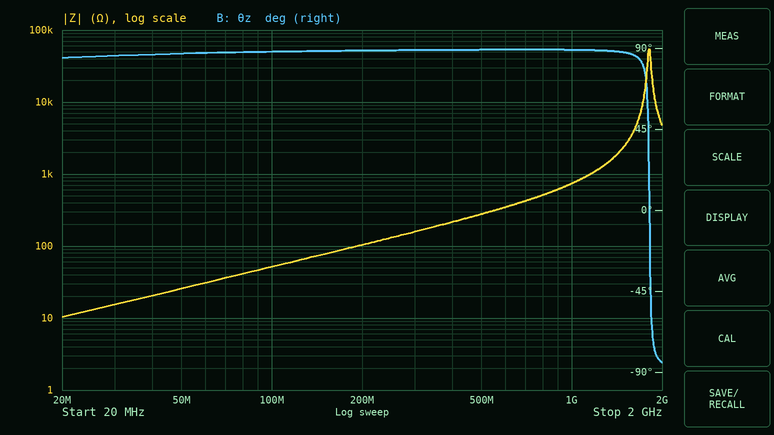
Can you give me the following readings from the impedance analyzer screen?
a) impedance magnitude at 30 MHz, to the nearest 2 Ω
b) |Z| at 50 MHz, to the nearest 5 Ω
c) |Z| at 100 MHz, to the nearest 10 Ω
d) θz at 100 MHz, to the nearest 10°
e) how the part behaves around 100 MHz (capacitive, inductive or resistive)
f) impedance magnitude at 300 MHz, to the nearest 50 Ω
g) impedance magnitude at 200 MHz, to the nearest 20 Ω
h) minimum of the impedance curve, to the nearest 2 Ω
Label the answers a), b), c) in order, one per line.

a) 16 Ω
b) 25 Ω
c) 50 Ω
d) 90°
e) inductive
f) 150 Ω
g) 100 Ω
h) 10 Ω
